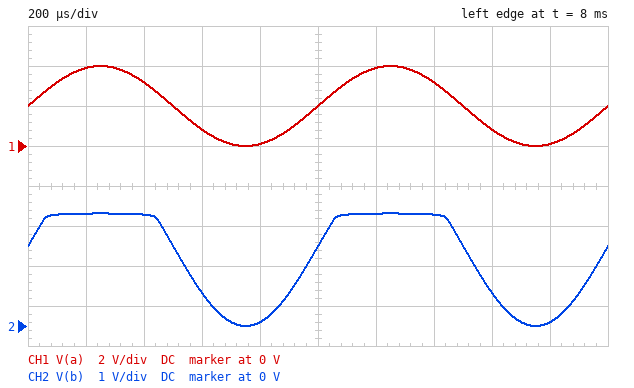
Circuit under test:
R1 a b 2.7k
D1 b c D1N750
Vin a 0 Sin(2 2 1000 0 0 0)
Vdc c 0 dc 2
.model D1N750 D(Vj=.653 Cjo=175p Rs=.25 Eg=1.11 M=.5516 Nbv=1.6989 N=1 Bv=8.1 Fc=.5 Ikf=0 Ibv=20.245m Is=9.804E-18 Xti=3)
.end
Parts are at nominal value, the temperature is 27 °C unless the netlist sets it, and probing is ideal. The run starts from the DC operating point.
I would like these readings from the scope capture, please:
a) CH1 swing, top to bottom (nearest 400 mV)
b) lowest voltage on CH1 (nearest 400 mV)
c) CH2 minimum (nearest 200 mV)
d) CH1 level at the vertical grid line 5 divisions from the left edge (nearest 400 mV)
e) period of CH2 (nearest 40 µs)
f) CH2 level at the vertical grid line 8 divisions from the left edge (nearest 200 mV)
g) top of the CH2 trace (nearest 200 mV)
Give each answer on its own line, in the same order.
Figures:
4.0 V
0 V
0 V
2.0 V
1.00 ms
800 mV
2.8 V
